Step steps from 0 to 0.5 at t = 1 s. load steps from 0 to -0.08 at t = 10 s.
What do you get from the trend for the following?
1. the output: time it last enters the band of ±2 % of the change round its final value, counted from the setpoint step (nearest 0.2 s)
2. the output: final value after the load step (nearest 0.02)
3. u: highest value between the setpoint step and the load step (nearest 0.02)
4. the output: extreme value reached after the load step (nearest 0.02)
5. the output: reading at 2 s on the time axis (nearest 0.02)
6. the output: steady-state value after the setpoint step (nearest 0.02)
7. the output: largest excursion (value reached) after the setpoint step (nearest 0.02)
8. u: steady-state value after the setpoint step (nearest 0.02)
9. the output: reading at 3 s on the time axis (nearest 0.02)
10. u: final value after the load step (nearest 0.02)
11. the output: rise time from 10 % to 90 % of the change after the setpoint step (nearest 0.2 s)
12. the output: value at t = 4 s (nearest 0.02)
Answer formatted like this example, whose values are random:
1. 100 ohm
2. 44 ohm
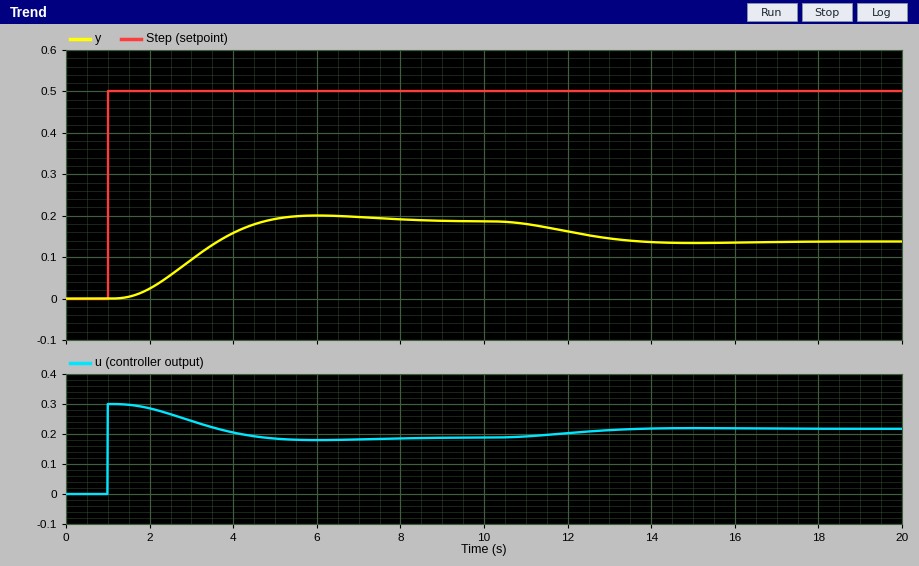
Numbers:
1. 7.0 s
2. 0.14
3. 0.30
4. 0.14
5. 0.02
6. 0.18
7. 0.20
8. 0.18
9. 0.10
10. 0.22
11. 2.4 s
12. 0.16
